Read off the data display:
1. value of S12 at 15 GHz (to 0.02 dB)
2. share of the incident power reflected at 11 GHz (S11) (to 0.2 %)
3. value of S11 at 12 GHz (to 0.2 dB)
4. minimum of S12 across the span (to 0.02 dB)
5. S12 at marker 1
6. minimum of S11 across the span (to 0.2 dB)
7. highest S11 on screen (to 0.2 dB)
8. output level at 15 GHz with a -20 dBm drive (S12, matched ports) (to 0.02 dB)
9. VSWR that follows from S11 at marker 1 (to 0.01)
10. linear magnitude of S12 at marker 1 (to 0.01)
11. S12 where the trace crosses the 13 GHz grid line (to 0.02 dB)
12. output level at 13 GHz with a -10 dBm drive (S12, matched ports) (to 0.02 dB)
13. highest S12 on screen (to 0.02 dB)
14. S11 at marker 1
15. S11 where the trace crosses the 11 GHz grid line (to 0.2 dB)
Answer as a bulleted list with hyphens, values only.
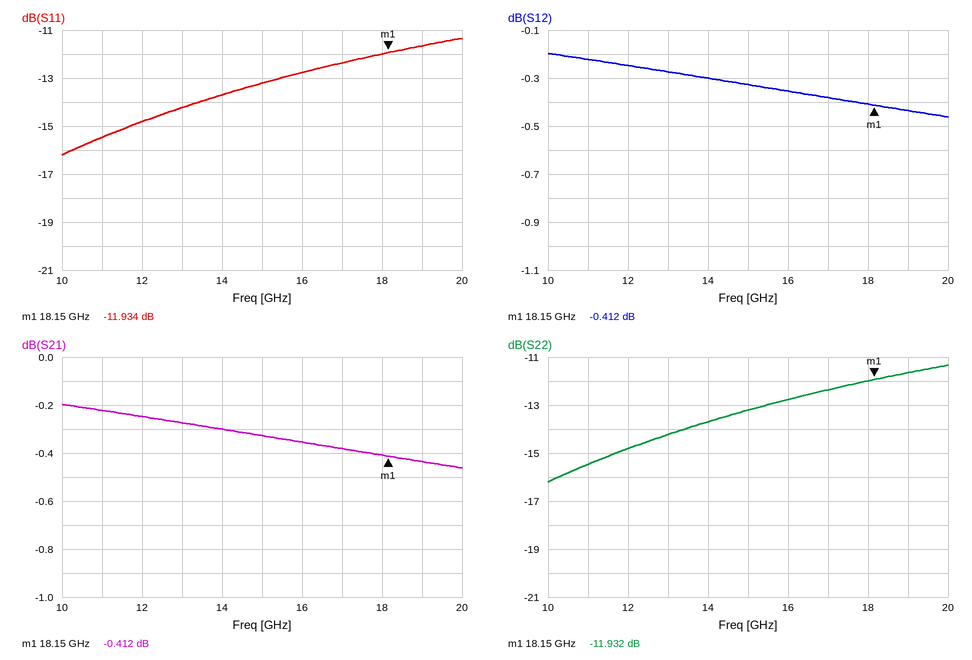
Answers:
- -0.32 dB
- 2.8 %
- -14.8 dB
- -0.46 dB
- -0.412 dB
- -16.2 dB
- -11.4 dB
- -20.32 dBm
- 1.68
- 0.95
- -0.28 dB
- -10.28 dBm
- -0.20 dB
- -11.934 dB
- -15.4 dB
